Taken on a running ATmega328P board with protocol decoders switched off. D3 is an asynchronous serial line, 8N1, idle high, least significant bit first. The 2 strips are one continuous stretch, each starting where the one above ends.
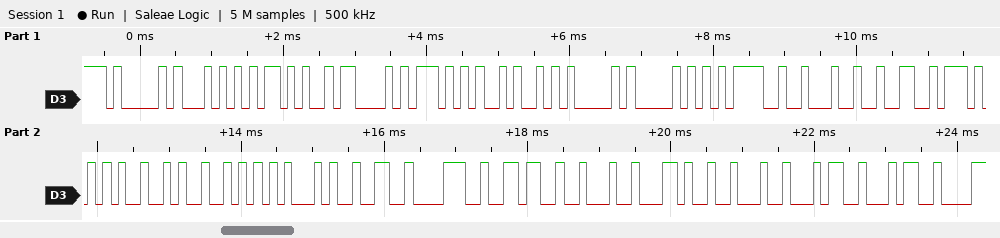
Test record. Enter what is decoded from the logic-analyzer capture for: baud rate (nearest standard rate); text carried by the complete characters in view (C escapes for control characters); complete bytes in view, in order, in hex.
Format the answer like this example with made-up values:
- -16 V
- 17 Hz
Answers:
- 9600 baud
- "AT+CWJAP=\"2WIRE286\",\"44"
- 0x41 0x54 0x2B 0x43 0x57 0x4A 0x41 0x50 0x3D 0x22 0x32 0x57 0x49 0x52 0x45 0x32 0x38 0x36 0x22 0x2C 0x22 0x34 0x34
